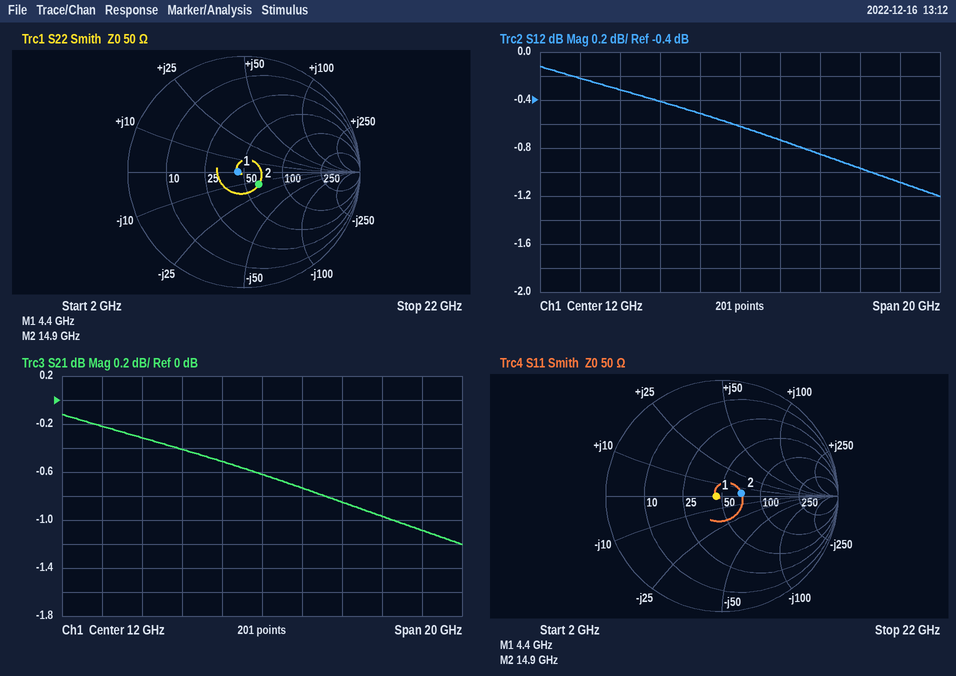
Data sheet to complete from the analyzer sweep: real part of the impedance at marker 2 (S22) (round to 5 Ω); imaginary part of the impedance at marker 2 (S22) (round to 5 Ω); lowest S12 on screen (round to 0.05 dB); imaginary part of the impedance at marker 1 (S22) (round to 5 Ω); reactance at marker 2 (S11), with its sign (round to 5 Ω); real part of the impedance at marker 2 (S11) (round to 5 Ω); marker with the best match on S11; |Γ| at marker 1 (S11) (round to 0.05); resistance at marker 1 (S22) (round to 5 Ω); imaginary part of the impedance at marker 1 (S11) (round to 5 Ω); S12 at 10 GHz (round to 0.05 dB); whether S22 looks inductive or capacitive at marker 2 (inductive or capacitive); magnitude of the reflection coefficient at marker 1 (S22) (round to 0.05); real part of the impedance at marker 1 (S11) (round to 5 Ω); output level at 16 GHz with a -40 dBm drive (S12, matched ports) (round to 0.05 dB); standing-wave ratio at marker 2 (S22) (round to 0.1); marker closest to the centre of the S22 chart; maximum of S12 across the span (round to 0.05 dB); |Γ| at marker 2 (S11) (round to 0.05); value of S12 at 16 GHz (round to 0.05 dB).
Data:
65 Ω
-15 Ω
-1.20 dB
0 Ω
+5 Ω
70 Ω
marker 1
0.05
45 Ω
0 Ω
-0.50 dB
capacitive
0.05
45 Ω
-40.85 dBm
1.4
marker 1
-0.10 dB
0.15
-0.85 dB
